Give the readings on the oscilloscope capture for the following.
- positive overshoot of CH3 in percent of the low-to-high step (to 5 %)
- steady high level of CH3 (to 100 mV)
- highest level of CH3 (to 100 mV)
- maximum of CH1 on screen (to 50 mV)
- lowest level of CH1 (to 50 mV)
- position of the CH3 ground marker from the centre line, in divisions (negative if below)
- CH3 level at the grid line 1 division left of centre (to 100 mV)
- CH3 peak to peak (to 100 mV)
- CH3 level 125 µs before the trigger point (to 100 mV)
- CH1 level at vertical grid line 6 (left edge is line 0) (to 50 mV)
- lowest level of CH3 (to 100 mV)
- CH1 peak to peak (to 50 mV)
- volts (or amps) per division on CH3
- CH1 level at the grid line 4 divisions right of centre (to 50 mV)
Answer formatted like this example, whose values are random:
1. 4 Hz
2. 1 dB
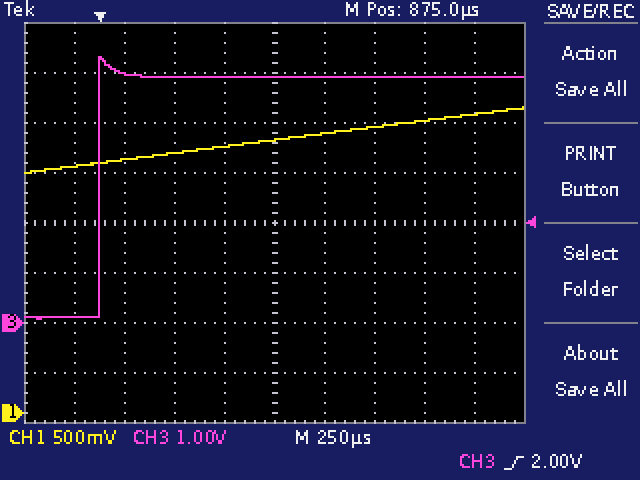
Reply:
1. 10 %
2. 4.9 V
3. 5.3 V
4. 3.05 V
5. 2.40 V
6. -2.0 div
7. 4.9 V
8. 5.2 V
9. 100 mV
10. 2.80 V
11. 100 mV
12. 650 mV
13. 1 V
14. 3.00 V
